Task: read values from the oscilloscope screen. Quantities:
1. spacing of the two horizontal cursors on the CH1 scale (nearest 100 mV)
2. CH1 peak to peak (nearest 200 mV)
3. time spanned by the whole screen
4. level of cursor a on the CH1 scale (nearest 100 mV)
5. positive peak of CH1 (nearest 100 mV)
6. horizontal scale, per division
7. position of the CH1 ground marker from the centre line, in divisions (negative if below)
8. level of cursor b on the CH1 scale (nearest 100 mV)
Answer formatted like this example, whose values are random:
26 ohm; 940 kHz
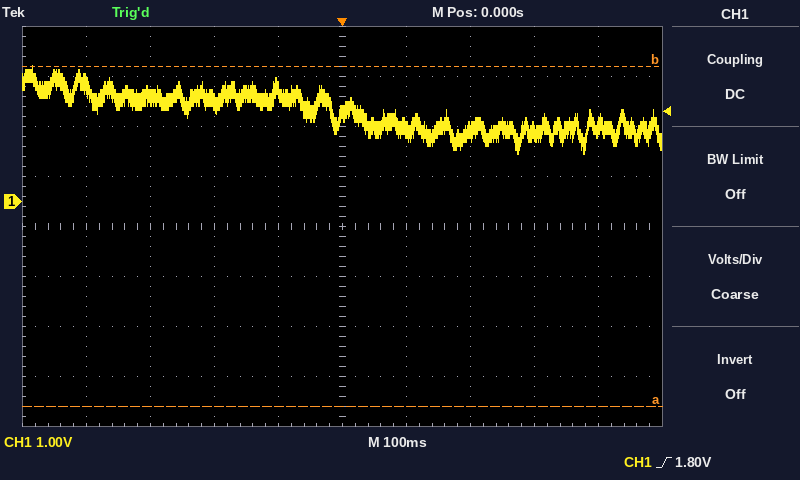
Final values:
6.8 V; 1.8 V; 1 s; -4.1 V; 2.7 V; 100 ms; +0.5 div; 2.7 V
